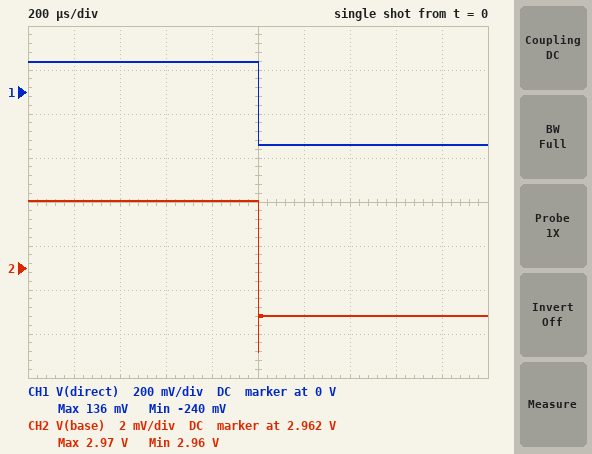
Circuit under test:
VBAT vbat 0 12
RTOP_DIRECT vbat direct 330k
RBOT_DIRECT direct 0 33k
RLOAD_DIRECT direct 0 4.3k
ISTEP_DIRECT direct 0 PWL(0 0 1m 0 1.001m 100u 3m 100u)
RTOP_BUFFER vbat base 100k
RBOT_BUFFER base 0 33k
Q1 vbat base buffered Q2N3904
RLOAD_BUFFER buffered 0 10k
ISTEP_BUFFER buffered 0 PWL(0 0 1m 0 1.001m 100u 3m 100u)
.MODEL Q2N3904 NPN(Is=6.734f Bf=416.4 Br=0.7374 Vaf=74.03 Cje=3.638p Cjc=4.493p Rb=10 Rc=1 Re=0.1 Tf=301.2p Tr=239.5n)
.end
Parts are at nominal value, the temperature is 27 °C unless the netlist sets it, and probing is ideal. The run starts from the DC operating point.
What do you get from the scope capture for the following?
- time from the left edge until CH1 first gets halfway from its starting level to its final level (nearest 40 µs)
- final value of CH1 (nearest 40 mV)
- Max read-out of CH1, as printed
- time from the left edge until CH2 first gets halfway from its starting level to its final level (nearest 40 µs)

1.00 ms
-240 mV
136 mV
1.00 ms
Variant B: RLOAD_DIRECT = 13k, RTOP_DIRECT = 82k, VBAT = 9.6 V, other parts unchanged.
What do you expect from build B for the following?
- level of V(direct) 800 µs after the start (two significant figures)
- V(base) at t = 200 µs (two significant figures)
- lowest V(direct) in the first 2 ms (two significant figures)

980 mV
2.4 V
140 mV
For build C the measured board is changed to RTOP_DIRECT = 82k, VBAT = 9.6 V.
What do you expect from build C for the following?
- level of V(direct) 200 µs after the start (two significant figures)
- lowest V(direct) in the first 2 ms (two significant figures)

430 mV
62 mV
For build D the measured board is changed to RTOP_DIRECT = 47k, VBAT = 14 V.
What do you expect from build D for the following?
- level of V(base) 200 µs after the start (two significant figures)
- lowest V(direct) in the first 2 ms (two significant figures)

3.5 V
700 mV
